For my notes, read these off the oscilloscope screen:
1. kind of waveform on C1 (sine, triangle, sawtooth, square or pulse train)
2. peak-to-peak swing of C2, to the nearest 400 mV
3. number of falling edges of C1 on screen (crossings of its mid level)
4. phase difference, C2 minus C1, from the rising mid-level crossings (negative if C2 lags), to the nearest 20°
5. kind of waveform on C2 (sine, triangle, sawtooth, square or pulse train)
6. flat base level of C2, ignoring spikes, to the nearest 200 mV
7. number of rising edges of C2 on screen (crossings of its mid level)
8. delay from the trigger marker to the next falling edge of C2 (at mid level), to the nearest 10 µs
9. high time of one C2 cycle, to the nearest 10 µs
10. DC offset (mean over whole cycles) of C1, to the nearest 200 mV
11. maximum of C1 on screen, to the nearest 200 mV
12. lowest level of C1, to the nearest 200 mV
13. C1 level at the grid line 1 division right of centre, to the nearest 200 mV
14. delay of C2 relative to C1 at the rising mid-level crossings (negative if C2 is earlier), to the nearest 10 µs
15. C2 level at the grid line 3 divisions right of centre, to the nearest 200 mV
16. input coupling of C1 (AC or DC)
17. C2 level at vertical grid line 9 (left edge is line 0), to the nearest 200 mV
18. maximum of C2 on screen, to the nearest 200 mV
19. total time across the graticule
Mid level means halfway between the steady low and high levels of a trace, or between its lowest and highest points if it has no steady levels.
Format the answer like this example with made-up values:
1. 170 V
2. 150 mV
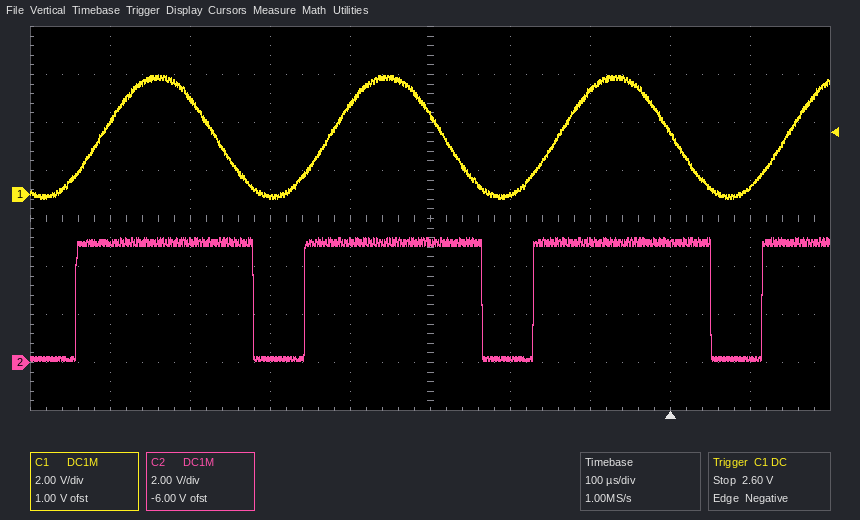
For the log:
1. sine
2. 5.2 V
3. 3
4. +40°
5. pulse train
6. 200 mV
7. 4
8. 50 µs
9. 220 µs
10. 2.4 V
11. 5.0 V
12. -200 mV
13. 0.0 V
14. -30 µs
15. 5.0 V
16. DC
17. 200 mV
18. 5.2 V
19. 1 ms
